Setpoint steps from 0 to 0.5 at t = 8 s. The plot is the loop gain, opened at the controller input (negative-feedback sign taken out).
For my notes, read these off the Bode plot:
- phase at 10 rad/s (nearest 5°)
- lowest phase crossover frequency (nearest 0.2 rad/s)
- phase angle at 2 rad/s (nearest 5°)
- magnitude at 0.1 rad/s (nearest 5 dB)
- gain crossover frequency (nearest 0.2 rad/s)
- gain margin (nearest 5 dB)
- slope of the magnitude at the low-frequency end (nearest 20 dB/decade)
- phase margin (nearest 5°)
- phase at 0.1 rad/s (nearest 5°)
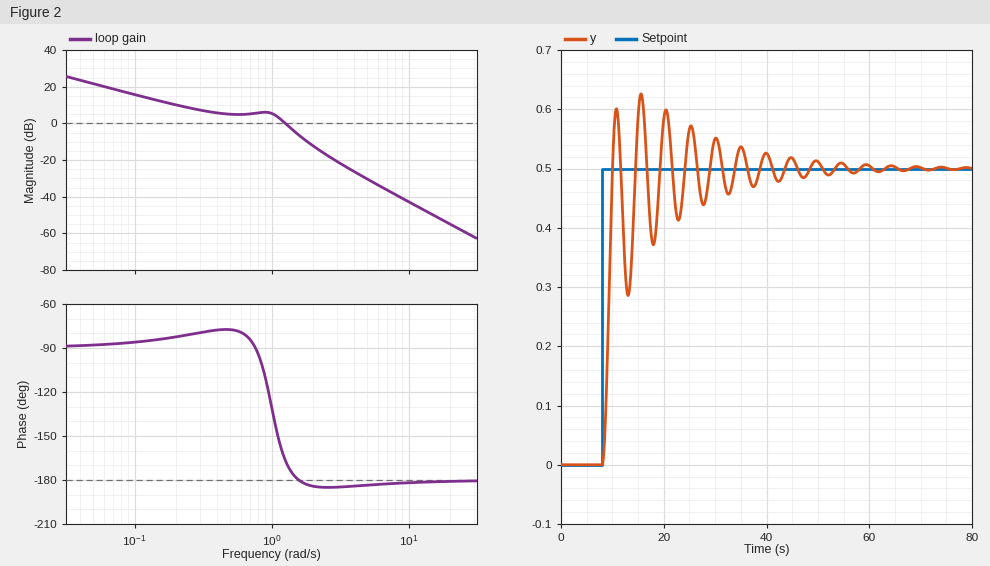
-180°
1.6 rad/s
-185°
15 dB
1.2 rad/s
5 dB
-20 dB/decade
15°
-85°
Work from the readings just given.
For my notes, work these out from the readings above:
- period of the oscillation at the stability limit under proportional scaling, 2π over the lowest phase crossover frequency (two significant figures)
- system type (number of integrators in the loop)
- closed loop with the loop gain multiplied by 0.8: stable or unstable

3.9 s
1
stable
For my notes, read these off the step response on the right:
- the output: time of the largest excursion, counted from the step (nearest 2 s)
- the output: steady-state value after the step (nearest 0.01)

8 s
0.50
